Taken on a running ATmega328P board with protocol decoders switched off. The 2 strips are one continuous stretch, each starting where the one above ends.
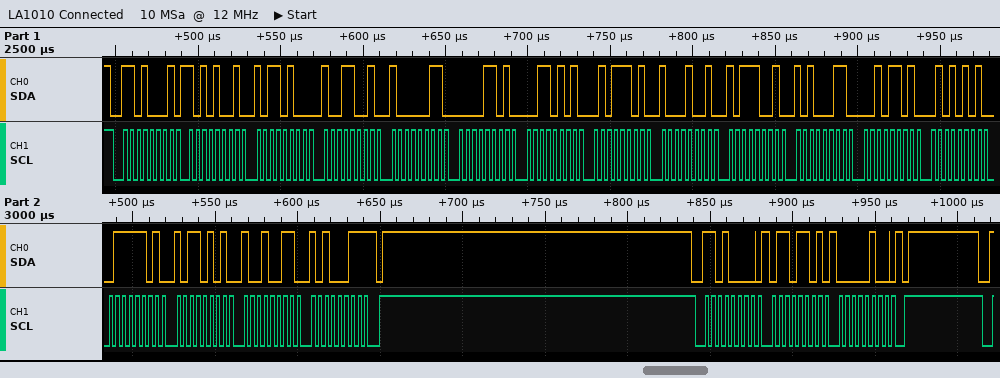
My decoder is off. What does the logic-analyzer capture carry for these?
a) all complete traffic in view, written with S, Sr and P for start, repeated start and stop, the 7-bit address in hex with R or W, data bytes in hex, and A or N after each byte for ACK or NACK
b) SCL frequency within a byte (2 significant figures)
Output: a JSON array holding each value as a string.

["S 68R A A9 A B4 A 99 A 83 A 0D A 35 A 5D A 89 A B9 A A3 A 2D A 55 A 7D A B5 A 93 A A3 N P S 68W A 6D A 04 A P", "250 kHz"]
